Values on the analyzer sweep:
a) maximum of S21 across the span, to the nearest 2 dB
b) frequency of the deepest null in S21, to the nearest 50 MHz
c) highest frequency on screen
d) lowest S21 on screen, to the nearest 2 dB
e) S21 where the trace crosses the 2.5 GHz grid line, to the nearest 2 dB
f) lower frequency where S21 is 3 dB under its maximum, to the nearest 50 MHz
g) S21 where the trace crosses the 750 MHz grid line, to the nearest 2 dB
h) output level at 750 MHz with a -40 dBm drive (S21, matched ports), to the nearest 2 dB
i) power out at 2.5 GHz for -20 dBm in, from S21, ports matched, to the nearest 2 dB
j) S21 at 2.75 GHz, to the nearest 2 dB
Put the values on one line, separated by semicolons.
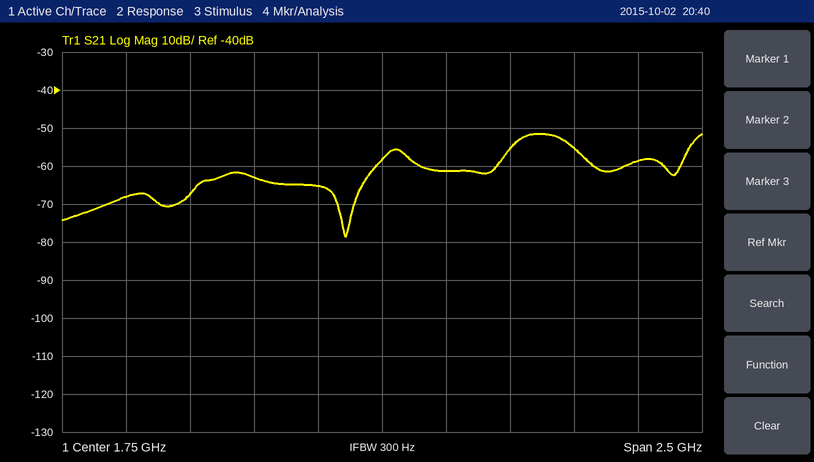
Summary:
-52 dB; 1.60 GHz; 3 GHz; -78 dB; -56 dB; 2.25 GHz; -68 dB; -108 dBm; -76 dBm; -58 dB
